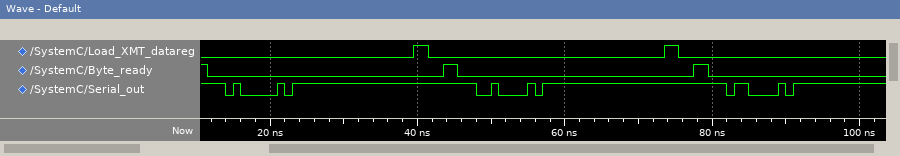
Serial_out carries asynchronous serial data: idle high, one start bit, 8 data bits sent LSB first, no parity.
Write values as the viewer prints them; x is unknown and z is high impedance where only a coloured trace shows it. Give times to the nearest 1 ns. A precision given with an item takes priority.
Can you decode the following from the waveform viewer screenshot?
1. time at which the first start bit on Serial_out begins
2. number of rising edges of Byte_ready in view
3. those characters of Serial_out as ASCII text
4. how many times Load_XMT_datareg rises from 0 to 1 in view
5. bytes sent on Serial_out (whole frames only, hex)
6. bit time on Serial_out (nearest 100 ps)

14 ns
2
"ABC"
2
41, 42, 43
1000 ps
